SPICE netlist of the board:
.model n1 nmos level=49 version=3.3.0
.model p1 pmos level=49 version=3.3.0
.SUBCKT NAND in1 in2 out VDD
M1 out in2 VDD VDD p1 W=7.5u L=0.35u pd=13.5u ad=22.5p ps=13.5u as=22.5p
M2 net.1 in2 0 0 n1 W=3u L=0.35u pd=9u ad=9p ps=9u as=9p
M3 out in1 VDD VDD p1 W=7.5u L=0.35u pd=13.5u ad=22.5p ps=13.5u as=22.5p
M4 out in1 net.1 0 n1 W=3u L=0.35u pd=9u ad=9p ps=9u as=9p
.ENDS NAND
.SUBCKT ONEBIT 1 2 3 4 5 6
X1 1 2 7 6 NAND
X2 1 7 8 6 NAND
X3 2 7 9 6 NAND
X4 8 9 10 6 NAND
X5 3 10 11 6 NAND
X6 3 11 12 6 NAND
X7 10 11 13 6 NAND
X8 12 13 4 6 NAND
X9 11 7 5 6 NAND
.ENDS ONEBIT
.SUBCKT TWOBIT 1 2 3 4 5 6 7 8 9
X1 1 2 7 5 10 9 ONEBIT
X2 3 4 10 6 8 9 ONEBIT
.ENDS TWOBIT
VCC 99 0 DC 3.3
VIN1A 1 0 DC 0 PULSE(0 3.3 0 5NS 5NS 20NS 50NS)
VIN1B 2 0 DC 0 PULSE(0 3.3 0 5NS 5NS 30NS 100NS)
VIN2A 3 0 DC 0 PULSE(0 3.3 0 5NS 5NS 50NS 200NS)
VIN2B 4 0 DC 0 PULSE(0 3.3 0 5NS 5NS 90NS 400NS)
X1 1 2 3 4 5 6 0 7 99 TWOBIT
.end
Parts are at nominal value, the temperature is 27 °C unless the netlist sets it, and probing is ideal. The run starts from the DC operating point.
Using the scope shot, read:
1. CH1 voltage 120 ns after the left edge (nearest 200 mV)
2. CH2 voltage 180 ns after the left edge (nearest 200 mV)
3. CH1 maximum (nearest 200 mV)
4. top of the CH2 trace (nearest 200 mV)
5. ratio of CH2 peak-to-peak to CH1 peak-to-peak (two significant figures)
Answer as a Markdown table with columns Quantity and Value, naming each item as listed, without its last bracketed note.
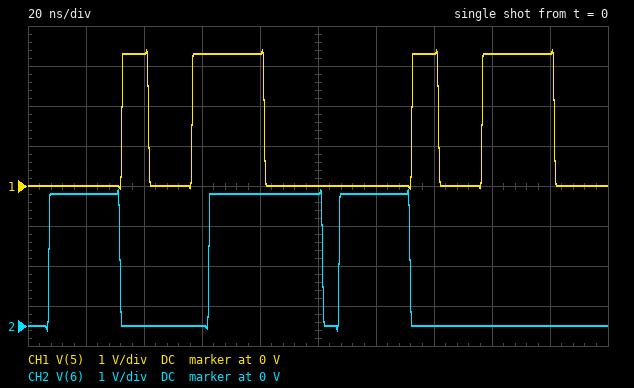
| Quantity | Value |
|---|---|
| CH1 voltage 120 ns after the left edge | 0 V |
| CH2 voltage 180 ns after the left edge | 0 V |
| CH1 maximum | 3.4 V |
| top of the CH2 trace | 3.4 V |
| ratio of CH2 peak-to-peak to CH1 peak-to-peak | 1.0 |
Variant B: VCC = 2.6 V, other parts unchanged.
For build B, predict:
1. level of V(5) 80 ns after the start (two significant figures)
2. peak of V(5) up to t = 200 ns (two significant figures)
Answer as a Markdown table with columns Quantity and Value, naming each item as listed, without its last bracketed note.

| Quantity | Value |
|---|---|
| level of V(5) 80 ns after the start | 2.6 V |
| peak of V(5) up to t = 200 ns | 2.7 V |
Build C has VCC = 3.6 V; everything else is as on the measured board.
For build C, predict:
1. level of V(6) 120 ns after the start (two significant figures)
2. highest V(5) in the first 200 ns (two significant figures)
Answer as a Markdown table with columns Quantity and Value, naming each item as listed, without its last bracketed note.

| Quantity | Value |
|---|---|
| level of V(6) 120 ns after the start | 3.6 V |
| highest V(5) in the first 200 ns | 3.7 V |
